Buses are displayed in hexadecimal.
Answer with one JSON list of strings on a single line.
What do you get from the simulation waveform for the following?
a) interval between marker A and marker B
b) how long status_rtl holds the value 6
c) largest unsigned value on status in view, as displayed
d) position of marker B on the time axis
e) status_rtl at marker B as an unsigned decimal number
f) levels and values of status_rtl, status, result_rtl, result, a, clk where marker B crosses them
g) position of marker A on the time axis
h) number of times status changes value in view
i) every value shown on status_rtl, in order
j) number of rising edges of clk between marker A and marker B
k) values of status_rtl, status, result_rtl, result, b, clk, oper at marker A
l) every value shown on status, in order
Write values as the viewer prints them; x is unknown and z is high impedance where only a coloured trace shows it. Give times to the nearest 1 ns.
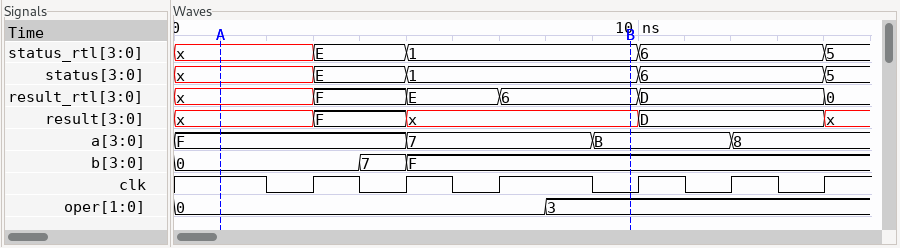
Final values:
["9 ns", "4 ns", "E", "10 ns", "1", "status_rtl=1, status=1, result_rtl=6, result=x, a=B, clk=0", "1 ns", "4", "x, E, 1, 6, 5", "3", "status_rtl=x, status=x, result_rtl=x, result=x, b=0, clk=1, oper=0", "x, E, 1, 6, 5"]
